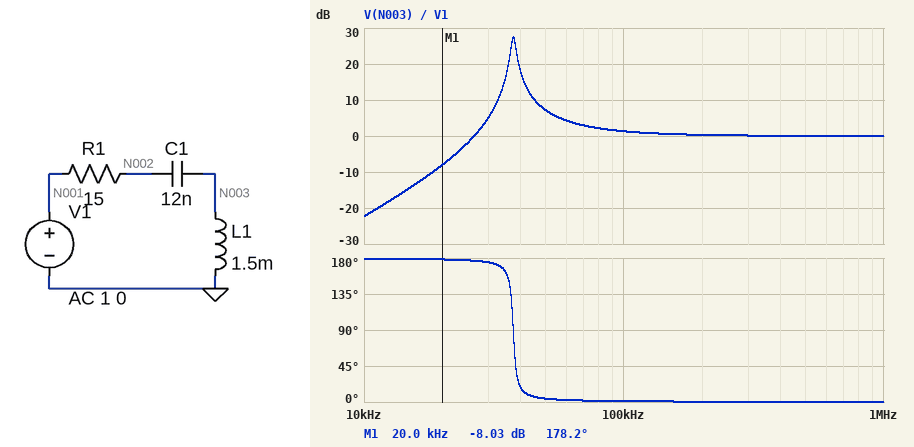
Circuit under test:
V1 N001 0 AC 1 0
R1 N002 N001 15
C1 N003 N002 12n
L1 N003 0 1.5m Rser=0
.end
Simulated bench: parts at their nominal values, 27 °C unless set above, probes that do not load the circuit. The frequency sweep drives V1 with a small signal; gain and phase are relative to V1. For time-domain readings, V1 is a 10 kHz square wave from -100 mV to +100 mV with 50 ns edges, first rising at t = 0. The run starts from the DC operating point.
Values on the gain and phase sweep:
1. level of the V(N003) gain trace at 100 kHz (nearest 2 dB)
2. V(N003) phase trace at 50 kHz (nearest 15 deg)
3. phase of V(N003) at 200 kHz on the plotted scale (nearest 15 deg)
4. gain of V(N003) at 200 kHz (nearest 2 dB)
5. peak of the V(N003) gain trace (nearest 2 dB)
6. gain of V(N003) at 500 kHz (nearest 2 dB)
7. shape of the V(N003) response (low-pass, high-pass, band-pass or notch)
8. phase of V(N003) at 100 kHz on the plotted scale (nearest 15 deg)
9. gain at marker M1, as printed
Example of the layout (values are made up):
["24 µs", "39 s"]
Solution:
["2 dB", "0 deg", "0 deg", "0 dB", "28 dB", "0 dB", "high-pass", "0 deg", "-8.03 dB"]
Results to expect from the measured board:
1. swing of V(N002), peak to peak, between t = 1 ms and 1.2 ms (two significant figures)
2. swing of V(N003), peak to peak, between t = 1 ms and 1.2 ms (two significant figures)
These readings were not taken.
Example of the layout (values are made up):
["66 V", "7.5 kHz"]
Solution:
["210 mV", "230 mV"]
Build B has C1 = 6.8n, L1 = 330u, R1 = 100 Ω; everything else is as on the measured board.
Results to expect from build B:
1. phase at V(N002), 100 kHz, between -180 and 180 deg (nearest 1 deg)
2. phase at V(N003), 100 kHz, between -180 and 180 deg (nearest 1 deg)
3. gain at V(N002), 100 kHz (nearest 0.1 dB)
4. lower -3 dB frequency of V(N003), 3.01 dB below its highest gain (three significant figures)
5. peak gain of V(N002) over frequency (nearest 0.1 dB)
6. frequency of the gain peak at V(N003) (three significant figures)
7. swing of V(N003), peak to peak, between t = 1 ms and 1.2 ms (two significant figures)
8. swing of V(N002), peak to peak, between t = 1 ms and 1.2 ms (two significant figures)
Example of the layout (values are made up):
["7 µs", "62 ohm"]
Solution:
["-75 deg", "105 deg", "-11.8 dB", "91.8 kHz", "0 dB", "112 kHz", "400 mV", "260 mV"]
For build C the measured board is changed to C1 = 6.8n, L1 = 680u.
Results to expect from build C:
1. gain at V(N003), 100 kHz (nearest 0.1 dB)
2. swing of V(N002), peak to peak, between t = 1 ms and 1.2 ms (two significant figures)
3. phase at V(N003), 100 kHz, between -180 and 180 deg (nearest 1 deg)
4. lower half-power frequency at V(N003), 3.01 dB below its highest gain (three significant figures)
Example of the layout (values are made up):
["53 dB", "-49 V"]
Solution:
["6.9 dB", "220 mV", "4 deg", "72.4 kHz"]
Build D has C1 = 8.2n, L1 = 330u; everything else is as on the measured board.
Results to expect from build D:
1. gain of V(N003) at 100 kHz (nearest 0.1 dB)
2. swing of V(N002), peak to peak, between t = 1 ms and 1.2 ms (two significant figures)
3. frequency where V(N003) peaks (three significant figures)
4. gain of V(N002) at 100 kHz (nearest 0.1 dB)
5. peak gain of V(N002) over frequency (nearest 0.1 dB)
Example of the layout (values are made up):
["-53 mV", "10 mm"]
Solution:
["20.3 dB", "220 mV", "96.9 kHz", "-3.6 dB", "0 dB"]
